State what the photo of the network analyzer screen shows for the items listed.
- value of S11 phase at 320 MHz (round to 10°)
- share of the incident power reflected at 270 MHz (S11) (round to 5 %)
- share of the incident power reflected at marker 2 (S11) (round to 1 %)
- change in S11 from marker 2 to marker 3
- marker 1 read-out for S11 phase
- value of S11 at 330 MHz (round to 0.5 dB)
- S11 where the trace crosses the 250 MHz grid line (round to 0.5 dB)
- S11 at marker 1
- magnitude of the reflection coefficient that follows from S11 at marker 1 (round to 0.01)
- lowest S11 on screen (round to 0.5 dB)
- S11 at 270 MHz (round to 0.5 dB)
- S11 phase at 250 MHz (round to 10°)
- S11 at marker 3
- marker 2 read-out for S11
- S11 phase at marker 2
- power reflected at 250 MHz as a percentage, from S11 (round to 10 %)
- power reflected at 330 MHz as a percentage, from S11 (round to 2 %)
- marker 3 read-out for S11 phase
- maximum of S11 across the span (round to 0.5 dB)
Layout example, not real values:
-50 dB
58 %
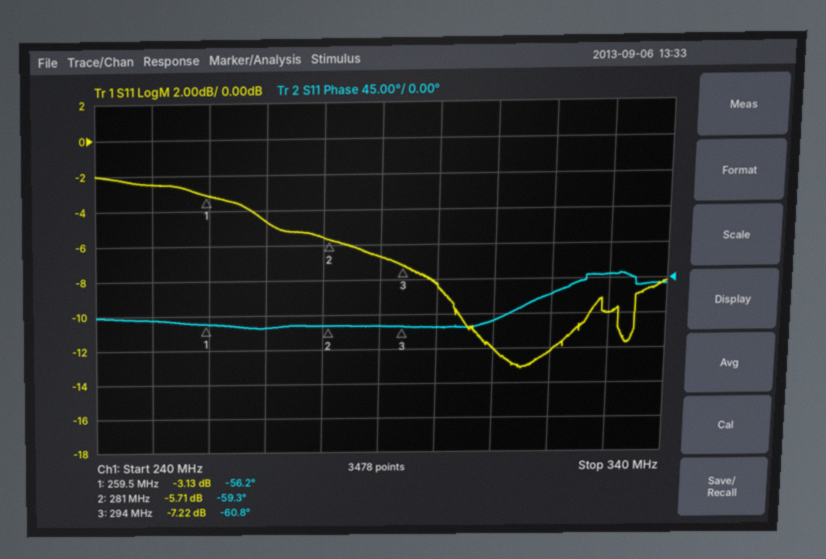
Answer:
-20°
35 %
27 %
-1.51 dB
-56.2°
-10.0 dB
-2.5 dB
-3.13 dB
0.70
-13.0 dB
-4.5 dB
-50°
-7.22 dB
-5.71 dB
-59.3°
60 %
10 %
-60.8°
-2.0 dB
